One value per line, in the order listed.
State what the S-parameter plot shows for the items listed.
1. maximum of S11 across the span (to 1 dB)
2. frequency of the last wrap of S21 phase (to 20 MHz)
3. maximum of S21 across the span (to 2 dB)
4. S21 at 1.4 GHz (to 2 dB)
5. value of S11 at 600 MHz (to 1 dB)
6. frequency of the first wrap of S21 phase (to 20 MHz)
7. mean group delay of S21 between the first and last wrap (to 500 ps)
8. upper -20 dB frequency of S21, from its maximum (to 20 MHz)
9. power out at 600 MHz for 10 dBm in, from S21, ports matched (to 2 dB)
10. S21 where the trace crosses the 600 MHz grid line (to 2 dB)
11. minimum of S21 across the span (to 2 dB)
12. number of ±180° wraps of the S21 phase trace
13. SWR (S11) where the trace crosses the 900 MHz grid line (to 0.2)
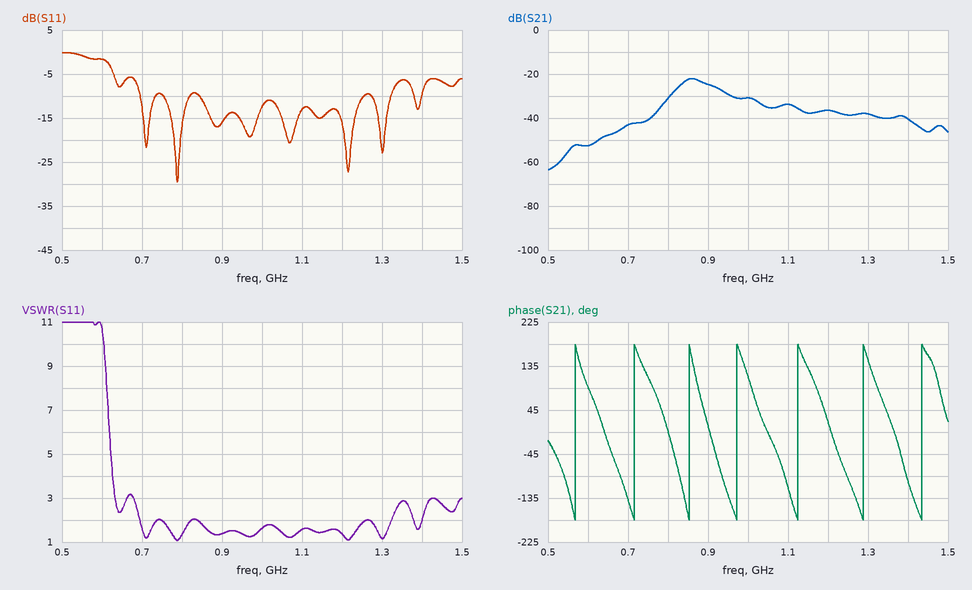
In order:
0 dB
1.44 GHz
-22 dB
-40 dB
-2 dB
560 MHz
7.0 ns
1.42 GHz
-42 dBm
-52 dB
-64 dB
7
1.4
